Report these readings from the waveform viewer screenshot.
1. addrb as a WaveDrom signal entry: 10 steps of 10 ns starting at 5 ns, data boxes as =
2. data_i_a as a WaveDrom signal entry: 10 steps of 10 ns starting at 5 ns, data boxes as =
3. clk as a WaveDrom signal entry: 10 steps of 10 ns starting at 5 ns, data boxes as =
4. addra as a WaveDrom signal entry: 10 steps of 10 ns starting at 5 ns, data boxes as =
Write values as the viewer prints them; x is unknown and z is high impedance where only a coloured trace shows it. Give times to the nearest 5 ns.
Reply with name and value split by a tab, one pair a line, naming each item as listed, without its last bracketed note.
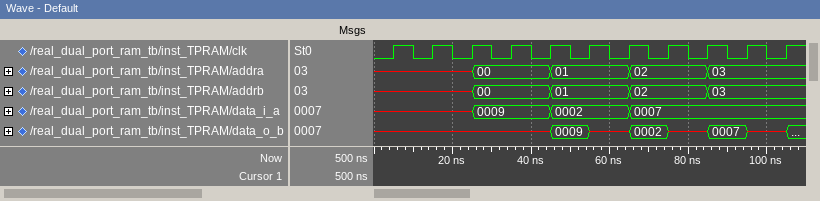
addrb as a WaveDrom signal entry: 10 steps of 10 ns starting at 5 ns, data boxes as =	{name: 'addrb', wave: 'x.=.=.=.=.', data: '00 01 02 03'}
data_i_a as a WaveDrom signal entry: 10 steps of 10 ns starting at 5 ns, data boxes as =	{name: 'data_i_a', wave: 'x.=.=.=...', data: '0009 0002 0007'}
clk as a WaveDrom signal entry: 10 steps of 10 ns starting at 5 ns, data boxes as =	{name: 'clk', wave: 'p.........'}
addra as a WaveDrom signal entry: 10 steps of 10 ns starting at 5 ns, data boxes as =	{name: 'addra', wave: 'x.=.=.=.=.', data: '00 01 02 03'}
